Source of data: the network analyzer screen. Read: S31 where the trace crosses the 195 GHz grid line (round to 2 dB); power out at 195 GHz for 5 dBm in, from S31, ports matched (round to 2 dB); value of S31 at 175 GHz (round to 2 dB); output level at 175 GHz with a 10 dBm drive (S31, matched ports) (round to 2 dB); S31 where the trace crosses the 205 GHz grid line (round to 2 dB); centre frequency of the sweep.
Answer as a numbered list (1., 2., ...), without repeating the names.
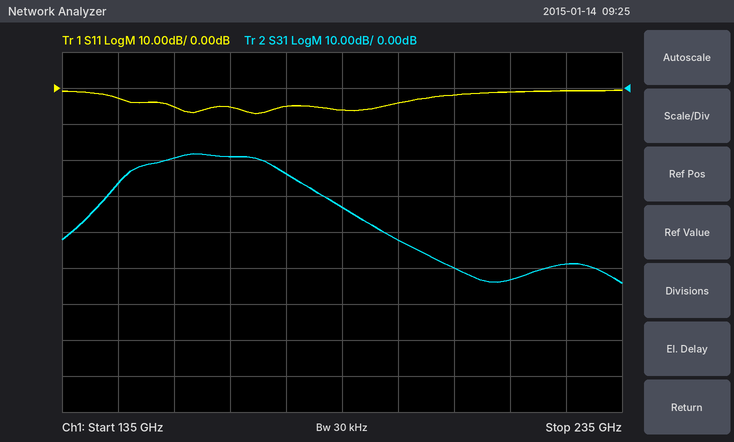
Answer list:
1. -42 dB
2. -38 dBm
3. -24 dB
4. -14 dBm
5. -50 dB
6. 185 GHz
